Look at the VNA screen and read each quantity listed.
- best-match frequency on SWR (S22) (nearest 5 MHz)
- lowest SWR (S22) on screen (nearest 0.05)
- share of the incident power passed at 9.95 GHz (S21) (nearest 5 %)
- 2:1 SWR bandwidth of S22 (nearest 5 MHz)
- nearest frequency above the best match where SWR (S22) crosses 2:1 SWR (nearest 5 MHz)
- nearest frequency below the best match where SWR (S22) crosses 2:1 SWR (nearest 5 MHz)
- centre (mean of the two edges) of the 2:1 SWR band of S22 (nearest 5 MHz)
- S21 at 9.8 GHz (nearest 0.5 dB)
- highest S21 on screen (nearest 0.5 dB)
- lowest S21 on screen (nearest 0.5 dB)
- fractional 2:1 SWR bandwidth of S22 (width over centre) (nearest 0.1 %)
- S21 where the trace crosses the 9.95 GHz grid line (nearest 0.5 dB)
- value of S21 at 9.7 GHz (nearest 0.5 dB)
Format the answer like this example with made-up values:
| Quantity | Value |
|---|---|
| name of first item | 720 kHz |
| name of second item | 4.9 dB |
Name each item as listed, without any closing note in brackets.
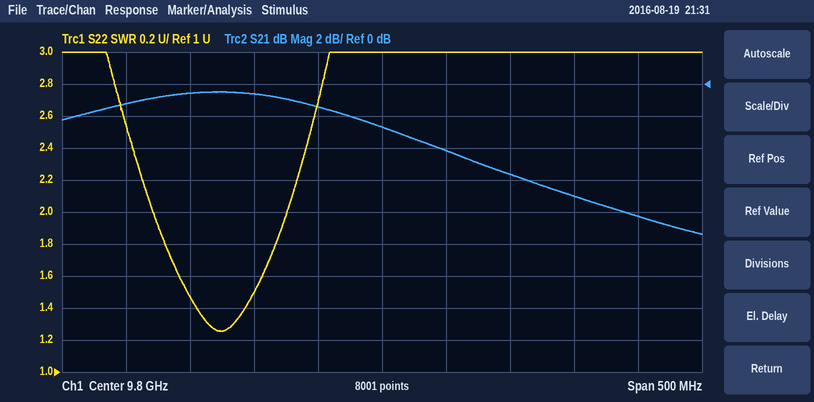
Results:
| Quantity | Value |
|---|---|
| best-match frequency on SWR (S22) | 9.675 GHz |
| lowest SWR (S22) on screen | 1.25 |
| share of the incident power passed at 9.95 GHz (S21) | 20 % |
| 2:1 SWR bandwidth of S22 | 105 MHz |
| nearest frequency above the best match where SWR (S22) crosses 2:1 SWR | 9.725 GHz |
| nearest frequency below the best match where SWR (S22) crosses 2:1 SWR | 9.620 GHz |
| centre (mean of the two edges) of the 2:1 SWR band of S22 | 9.675 GHz |
| S21 at 9.8 GHz | -2.5 dB |
| highest S21 on screen | -0.5 dB |
| lowest S21 on screen | -9.5 dB |
| fractional 2:1 SWR bandwidth of S22 (width over centre) | 1.1 % |
| S21 where the trace crosses the 9.95 GHz grid line | -7.0 dB |
| value of S21 at 9.7 GHz | -0.5 dB |
